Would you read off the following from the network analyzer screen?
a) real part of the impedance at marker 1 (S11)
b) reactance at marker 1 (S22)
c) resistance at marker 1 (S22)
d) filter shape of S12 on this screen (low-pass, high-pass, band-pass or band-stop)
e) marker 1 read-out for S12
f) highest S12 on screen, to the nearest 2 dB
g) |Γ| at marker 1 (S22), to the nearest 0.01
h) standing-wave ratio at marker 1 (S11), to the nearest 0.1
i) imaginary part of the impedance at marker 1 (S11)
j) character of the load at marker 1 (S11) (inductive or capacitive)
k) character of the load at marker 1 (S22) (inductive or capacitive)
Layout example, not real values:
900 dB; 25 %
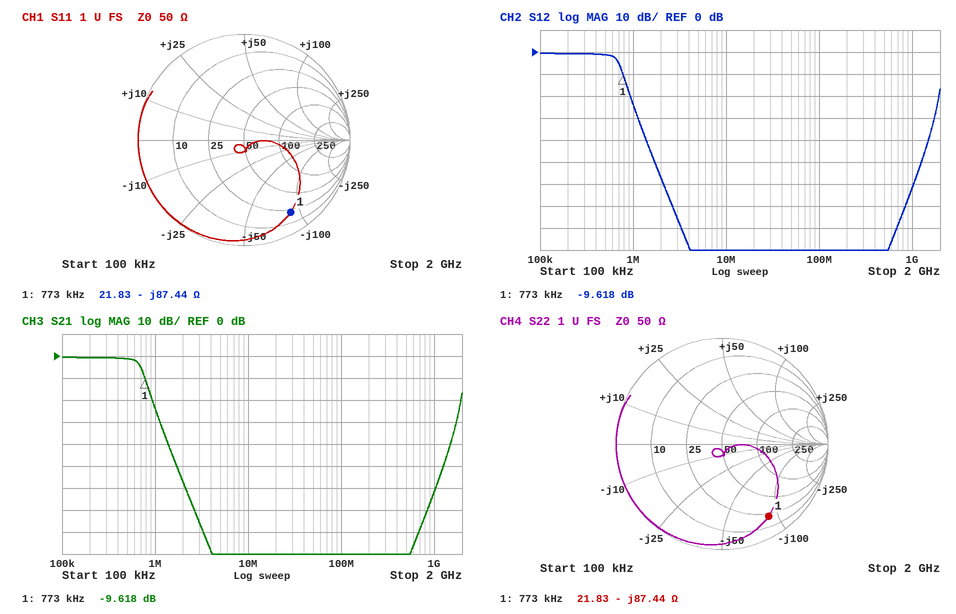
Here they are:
21.83 Ω; -87.44 Ω; 21.83 Ω; low-pass; -9.618 dB; 0 dB; 0.81; 9.6; -87.44 Ω; capacitive; capacitive
